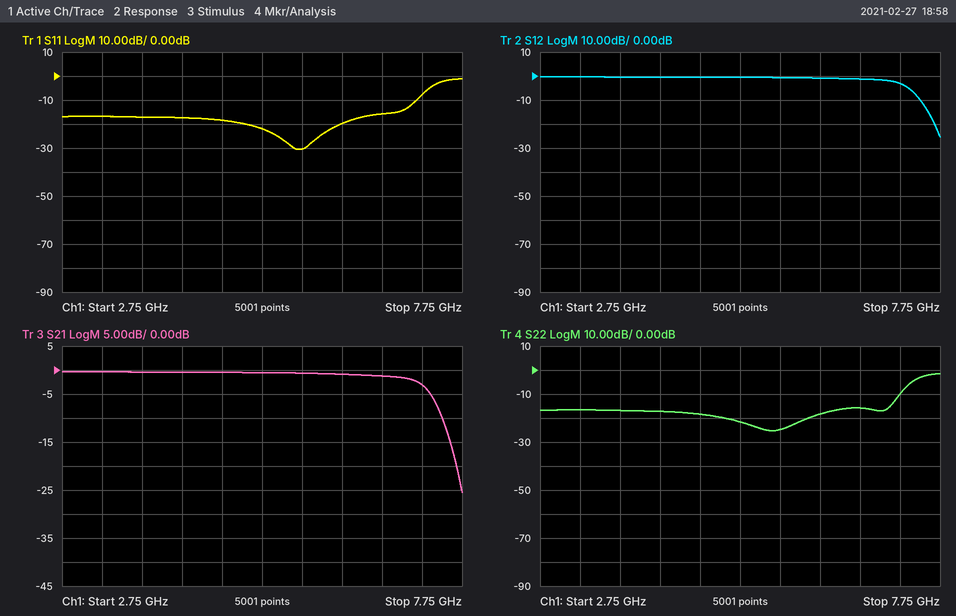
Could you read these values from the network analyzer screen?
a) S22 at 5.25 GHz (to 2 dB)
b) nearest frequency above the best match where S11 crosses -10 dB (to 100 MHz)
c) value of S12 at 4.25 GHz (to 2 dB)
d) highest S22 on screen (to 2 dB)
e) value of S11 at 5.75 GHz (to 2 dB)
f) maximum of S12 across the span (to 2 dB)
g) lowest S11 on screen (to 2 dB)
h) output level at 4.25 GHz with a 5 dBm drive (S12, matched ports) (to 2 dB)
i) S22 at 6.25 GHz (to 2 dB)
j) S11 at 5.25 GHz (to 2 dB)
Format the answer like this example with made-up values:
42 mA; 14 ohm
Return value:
-22 dB; 7.2 GHz; 0 dB; -2 dB; -30 dB; 0 dB; -30 dB; 4 dBm; -18 dB; -22 dB
